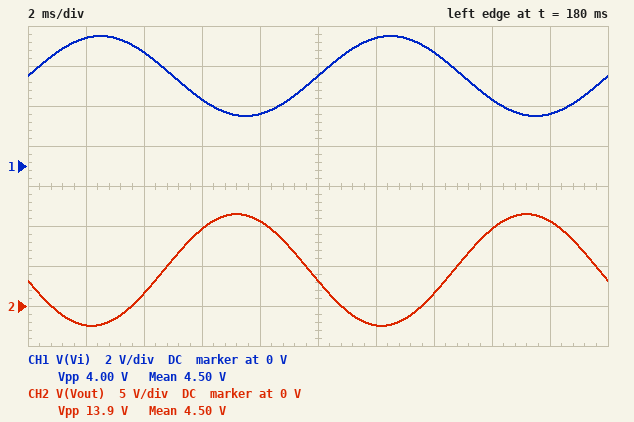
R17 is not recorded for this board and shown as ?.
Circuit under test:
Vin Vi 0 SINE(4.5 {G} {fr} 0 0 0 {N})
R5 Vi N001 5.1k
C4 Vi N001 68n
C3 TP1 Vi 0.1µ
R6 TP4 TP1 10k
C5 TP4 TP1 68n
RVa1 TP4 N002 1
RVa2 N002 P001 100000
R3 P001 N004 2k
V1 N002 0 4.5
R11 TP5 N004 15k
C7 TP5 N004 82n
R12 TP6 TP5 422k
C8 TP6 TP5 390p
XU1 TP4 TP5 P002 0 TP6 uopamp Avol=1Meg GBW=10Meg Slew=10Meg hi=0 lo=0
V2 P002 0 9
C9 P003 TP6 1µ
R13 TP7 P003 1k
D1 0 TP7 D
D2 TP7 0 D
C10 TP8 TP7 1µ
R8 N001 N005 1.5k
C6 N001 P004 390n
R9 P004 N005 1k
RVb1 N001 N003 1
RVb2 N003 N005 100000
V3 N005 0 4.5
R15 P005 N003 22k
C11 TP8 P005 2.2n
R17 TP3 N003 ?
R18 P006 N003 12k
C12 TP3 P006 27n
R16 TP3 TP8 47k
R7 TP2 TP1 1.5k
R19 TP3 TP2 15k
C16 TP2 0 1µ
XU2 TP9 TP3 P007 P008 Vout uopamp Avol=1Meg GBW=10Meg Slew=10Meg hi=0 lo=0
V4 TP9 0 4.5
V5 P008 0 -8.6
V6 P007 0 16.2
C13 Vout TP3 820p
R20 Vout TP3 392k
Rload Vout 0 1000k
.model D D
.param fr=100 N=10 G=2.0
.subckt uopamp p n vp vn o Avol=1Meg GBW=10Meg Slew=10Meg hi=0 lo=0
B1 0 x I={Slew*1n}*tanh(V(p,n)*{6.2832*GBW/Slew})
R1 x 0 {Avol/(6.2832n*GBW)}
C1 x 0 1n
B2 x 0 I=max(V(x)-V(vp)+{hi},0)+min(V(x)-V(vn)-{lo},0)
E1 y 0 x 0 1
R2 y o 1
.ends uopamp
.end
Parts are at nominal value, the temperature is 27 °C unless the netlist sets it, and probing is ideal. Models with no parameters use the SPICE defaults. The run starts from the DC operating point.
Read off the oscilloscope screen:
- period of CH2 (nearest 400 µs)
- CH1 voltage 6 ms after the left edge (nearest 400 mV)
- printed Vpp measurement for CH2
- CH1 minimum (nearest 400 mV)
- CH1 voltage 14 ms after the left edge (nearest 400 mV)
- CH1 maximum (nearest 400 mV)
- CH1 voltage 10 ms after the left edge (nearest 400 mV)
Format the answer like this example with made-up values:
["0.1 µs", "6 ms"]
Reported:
["10.0 ms", "3.2 V", "13.9 V", "2.4 V", "5.6 V", "6.4 V", "4.4 V"]
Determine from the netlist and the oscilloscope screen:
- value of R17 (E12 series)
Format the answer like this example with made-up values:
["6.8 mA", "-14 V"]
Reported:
["82 kΩ"]
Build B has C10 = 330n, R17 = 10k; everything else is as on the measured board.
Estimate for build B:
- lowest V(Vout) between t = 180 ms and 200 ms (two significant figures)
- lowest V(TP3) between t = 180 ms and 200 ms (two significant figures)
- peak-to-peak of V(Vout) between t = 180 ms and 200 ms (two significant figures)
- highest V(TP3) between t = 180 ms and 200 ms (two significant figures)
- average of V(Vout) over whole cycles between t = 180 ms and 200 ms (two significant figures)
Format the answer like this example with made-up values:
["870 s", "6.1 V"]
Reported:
["-8.6 V", "4.4 V", "25 V", "4.6 V", "4.2 V"]
